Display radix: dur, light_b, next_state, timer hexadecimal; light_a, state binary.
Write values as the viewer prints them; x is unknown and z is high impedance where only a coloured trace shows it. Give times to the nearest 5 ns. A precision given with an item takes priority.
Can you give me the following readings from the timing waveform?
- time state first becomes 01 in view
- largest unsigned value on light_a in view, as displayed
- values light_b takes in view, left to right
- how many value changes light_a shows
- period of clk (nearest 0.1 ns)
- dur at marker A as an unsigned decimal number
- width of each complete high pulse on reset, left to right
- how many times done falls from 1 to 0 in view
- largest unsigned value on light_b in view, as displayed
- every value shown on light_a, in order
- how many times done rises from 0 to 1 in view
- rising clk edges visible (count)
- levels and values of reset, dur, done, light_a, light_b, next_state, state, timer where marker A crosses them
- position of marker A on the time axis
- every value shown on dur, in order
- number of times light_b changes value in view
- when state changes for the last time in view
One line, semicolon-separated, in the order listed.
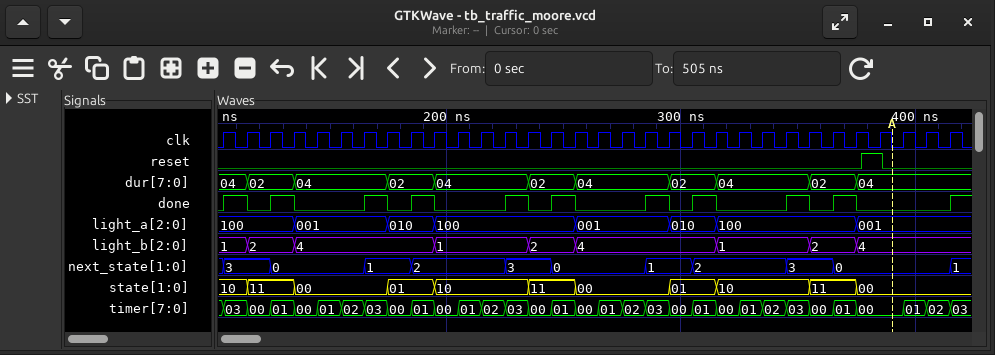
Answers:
175 ns; 100; 1, 2, 4, 1, 2, 4, 1, 2, 4; 7; 10 ns; 4; 10 ns; 10; 4; 100, 001, 010, 100, 001, 010, 100, 001; 11; 32; reset=0, dur=04, done=0, light_a=001, light_b=4, next_state=0, state=00, timer=00; 390 ns; 04, 02, 04, 02, 04, 02, 04, 02, 04, 02, 04; 8; 375 ns
